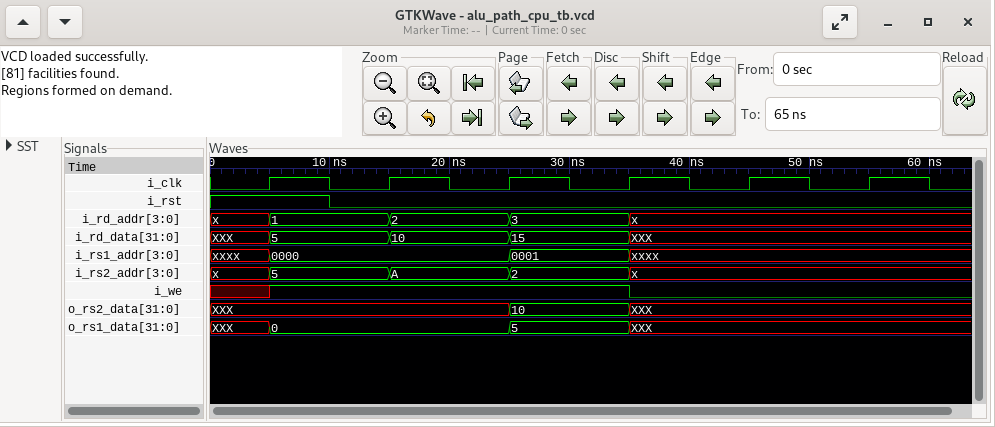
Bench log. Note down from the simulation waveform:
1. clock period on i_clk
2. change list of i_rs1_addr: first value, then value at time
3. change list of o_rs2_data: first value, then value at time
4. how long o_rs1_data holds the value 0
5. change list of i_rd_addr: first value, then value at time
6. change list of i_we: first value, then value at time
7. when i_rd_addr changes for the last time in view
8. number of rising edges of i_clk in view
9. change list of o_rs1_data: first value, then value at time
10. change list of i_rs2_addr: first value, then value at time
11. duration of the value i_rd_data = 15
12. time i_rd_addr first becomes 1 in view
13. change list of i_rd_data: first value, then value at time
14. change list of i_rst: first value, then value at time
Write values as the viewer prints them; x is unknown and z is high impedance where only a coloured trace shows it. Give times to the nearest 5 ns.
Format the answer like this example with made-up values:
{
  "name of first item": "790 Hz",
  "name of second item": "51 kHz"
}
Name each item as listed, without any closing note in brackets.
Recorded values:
{
  "clock period on i_clk": "10 ns",
  "change list of i_rs1_addr: first value, then value at time": "xxxx, 0000 at 5 ns, 0001 at 25 ns, xxxx at 35 ns",
  "change list of o_rs2_data: first value, then value at time": "XXX, 10 at 25 ns, XXX at 35 ns",
  "how long o_rs1_data holds the value 0": "20 ns",
  "change list of i_rd_addr: first value, then value at time": "x, 1 at 5 ns, 2 at 15 ns, 3 at 25 ns, x at 35 ns",
  "change list of i_we: first value, then value at time": "x, 1 at 5 ns, 0 at 35 ns",
  "when i_rd_addr changes for the last time in view": "35 ns",
  "number of rising edges of i_clk in view": "6",
  "change list of o_rs1_data: first value, then value at time": "XXX, 0 at 5 ns, 5 at 25 ns, XXX at 35 ns",
  "change list of i_rs2_addr: first value, then value at time": "x, 5 at 5 ns, A at 15 ns, 2 at 25 ns, x at 35 ns",
  "duration of the value i_rd_data = 15": "10 ns",
  "time i_rd_addr first becomes 1 in view": "5 ns",
  "change list of i_rd_data: first value, then value at time": "XXX, 5 at 5 ns, 10 at 15 ns, 15 at 25 ns, XXX at 35 ns",
  "change list of i_rst: first value, then value at time": "1, 0 at 10 ns"
}
